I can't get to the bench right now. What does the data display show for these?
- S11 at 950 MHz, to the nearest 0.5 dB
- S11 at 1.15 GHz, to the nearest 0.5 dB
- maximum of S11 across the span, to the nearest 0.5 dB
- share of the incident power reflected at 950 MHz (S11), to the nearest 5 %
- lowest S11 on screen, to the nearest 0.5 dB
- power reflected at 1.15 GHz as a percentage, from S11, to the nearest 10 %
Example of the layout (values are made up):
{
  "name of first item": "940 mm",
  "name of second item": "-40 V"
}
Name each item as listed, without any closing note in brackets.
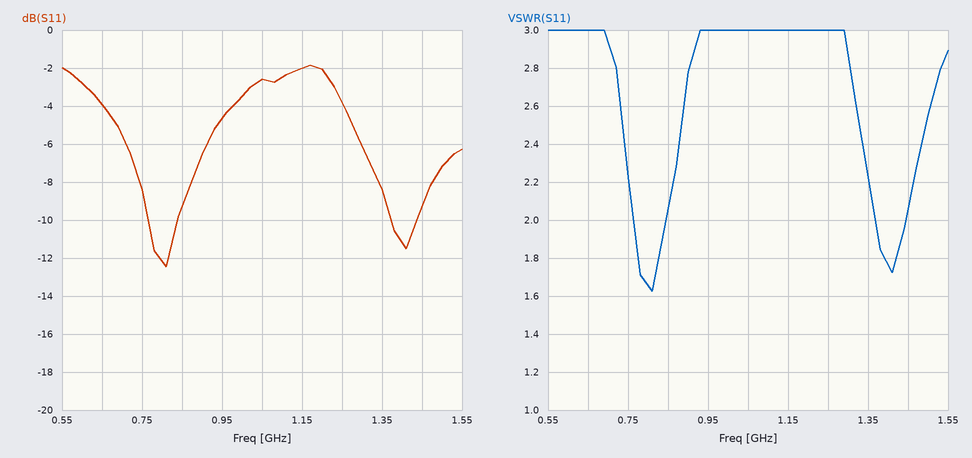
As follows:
{
  "S11 at 950 MHz, to the nearest 0.5 dB": "-4.5 dB",
  "S11 at 1.15 GHz, to the nearest 0.5 dB": "-2.0 dB",
  "maximum of S11 across the span, to the nearest 0.5 dB": "-2.0 dB",
  "share of the incident power reflected at 950 MHz (S11), to the nearest 5 %": "35 %",
  "lowest S11 on screen, to the nearest 0.5 dB": "-12.5 dB",
  "power reflected at 1.15 GHz as a percentage, from S11, to the nearest 10 %": "60 %"
}
